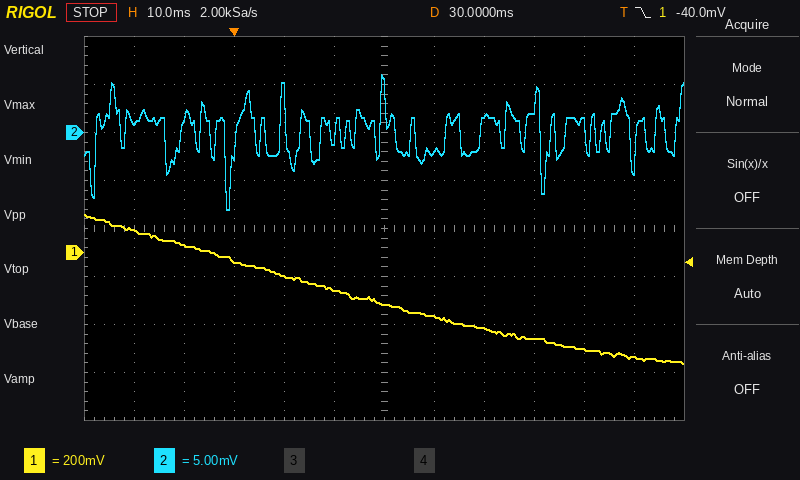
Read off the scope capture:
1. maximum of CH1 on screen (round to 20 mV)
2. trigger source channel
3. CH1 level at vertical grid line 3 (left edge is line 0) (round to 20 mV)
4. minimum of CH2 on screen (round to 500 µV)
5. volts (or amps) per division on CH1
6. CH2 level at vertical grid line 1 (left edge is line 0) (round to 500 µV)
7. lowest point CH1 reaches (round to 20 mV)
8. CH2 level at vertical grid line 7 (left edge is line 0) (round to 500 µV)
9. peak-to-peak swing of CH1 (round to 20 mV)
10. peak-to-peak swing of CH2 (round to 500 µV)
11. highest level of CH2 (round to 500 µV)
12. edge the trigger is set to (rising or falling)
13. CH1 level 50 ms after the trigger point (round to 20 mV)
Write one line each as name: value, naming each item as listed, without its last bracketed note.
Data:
maximum of CH1 on screen: 160 mV
trigger source channel: CH1
CH1 level at vertical grid line 3 (left edge is line 0): -40 mV
minimum of CH2 on screen: -8.0 mV
volts (or amps) per division on CH1: 200 mV
CH2 level at vertical grid line 1 (left edge is line 0): 1.0 mV
lowest point CH1 reaches: -460 mV
CH2 level at vertical grid line 7 (left edge is line 0): -2.0 mV
peak-to-peak swing of CH1: 620 mV
peak-to-peak swing of CH2: 14.0 mV
highest level of CH2: 6.0 mV
edge the trigger is set to: falling
CH1 level 50 ms after the trigger point: -320 mV
